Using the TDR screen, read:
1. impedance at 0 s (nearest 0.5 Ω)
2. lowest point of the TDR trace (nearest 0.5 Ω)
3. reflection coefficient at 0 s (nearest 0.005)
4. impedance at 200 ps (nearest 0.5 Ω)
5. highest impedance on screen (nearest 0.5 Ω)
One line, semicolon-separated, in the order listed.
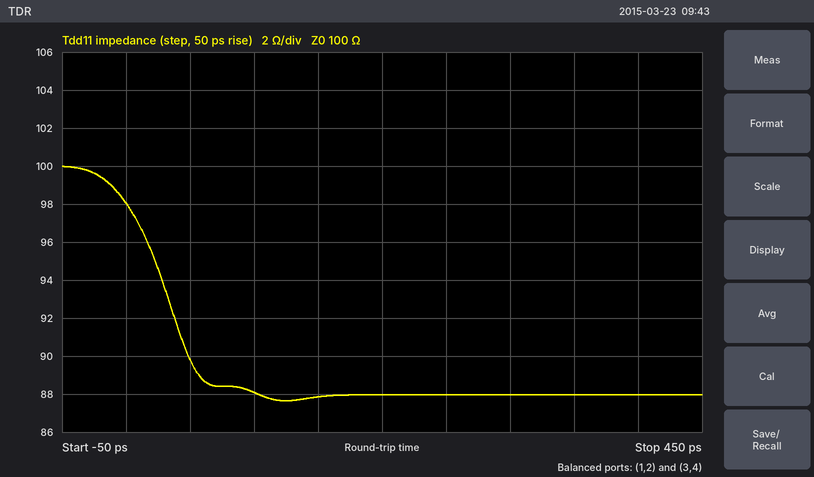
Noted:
98.0 Ω; 87.5 Ω; -0.010; 88.0 Ω; 100.0 Ω
